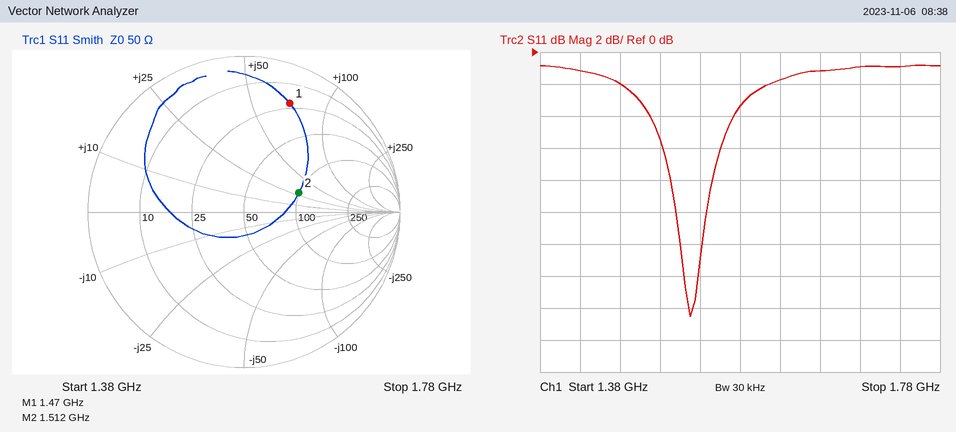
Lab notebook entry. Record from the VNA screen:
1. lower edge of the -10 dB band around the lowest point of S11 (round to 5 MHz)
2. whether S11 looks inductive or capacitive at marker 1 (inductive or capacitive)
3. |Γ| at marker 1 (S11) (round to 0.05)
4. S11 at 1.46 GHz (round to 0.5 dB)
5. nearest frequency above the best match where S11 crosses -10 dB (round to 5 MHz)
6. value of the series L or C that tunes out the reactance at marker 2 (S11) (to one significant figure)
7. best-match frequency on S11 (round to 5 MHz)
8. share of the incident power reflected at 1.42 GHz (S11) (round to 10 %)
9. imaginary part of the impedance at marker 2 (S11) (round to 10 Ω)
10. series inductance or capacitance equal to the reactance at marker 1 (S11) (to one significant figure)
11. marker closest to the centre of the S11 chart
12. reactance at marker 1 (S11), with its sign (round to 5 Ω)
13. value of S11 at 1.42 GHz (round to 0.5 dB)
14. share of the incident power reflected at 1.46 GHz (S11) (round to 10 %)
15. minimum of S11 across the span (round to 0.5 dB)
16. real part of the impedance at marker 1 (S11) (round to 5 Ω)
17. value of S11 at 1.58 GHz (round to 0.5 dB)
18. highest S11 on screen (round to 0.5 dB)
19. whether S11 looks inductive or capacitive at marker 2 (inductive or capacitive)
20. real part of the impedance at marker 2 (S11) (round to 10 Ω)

1.515 GHz
inductive
0.75
-2.0 dB
1.545 GHz
4 pF
1.530 GHz
80 %
+30 Ω
8 nH
marker 2
+70 Ω
-1.0 dB
60 %
-16.5 dB
20 Ω
-3.5 dB
-1.0 dB
inductive
100 Ω
